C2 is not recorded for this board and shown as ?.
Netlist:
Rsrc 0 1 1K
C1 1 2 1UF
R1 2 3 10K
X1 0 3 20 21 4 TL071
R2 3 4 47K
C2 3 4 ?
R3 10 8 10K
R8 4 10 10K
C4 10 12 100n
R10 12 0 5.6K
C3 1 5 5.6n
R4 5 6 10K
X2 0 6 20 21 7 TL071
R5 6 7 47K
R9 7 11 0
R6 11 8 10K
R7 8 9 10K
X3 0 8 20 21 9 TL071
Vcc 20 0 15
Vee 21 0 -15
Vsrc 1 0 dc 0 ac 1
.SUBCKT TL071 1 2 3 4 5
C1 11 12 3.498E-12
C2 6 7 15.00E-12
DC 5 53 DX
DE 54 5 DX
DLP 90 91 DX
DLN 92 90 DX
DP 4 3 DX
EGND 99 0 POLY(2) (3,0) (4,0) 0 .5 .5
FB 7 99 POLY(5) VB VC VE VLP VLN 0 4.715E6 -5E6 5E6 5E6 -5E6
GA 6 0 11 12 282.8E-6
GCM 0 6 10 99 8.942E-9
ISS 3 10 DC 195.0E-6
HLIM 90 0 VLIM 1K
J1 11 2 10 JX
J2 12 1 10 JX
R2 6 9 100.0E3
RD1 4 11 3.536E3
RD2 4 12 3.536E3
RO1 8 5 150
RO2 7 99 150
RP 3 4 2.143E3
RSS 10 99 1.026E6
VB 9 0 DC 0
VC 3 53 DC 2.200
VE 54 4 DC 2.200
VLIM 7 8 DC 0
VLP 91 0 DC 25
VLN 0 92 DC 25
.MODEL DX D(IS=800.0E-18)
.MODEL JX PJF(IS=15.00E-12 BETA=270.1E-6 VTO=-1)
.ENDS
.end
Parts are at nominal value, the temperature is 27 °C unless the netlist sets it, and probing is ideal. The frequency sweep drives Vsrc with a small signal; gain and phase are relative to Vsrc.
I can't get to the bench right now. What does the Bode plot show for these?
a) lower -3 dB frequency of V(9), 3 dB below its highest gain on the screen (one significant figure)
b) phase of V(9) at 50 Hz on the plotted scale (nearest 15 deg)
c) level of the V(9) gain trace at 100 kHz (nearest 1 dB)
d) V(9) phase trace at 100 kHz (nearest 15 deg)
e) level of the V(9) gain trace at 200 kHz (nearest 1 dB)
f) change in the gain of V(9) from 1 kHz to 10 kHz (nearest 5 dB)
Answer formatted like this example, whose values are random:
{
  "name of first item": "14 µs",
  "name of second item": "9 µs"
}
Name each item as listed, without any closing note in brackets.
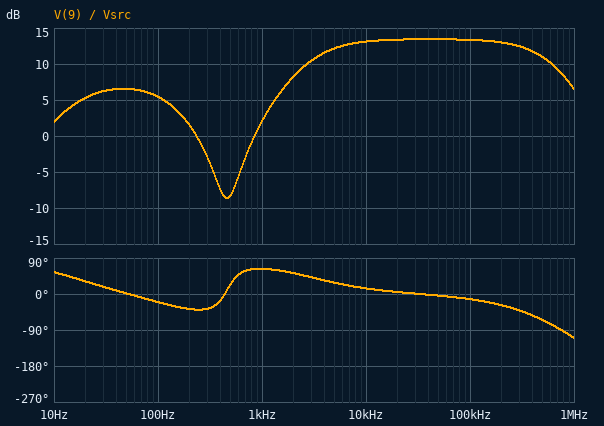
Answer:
{
  "lower -3 dB frequency of V(9), 3 dB below its highest gain on the screen": "3 kHz",
  "phase of V(9) at 50 Hz on the plotted scale": "0 deg",
  "level of the V(9) gain trace at 100 kHz": "13 dB",
  "V(9) phase trace at 100 kHz": "-15 deg",
  "level of the V(9) gain trace at 200 kHz": "13 dB",
  "change in the gain of V(9) from 1 kHz to 10 kHz": "10 dB"
}
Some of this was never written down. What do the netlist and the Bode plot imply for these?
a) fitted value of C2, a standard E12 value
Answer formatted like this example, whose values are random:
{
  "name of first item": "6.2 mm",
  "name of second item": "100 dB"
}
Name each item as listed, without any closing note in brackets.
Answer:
{
  "fitted value of C2, a standard E12 value": "12 nF"
}
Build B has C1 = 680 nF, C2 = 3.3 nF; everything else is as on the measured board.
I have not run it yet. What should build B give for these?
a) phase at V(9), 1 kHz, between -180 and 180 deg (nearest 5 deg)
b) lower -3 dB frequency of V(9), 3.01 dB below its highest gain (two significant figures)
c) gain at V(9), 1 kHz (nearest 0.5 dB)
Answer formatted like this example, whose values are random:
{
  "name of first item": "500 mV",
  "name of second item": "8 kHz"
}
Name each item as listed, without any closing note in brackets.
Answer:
{
  "phase at V(9), 1 kHz, between -180 and 180 deg": "35 deg",
  "lower -3 dB frequency of V(9), 3.01 dB below its highest gain": "3.1 kHz",
  "gain at V(9), 1 kHz": "2.5 dB"
}
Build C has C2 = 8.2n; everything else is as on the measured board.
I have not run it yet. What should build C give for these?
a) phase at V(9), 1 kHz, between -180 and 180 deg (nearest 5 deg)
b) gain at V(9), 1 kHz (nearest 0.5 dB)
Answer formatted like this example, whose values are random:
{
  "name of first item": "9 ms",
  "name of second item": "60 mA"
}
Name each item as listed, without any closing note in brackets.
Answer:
{
  "phase at V(9), 1 kHz, between -180 and 180 deg": "55 deg",
  "gain at V(9), 1 kHz": "1.5 dB"
}
